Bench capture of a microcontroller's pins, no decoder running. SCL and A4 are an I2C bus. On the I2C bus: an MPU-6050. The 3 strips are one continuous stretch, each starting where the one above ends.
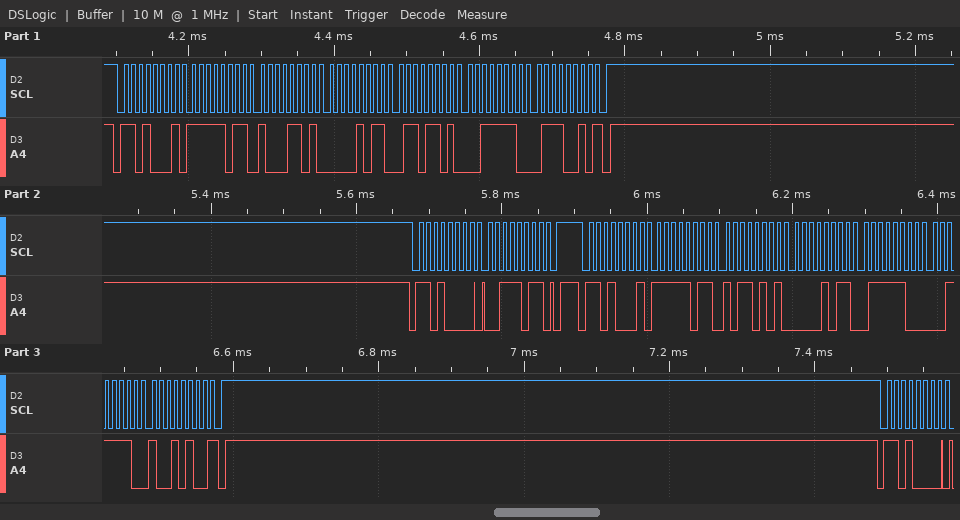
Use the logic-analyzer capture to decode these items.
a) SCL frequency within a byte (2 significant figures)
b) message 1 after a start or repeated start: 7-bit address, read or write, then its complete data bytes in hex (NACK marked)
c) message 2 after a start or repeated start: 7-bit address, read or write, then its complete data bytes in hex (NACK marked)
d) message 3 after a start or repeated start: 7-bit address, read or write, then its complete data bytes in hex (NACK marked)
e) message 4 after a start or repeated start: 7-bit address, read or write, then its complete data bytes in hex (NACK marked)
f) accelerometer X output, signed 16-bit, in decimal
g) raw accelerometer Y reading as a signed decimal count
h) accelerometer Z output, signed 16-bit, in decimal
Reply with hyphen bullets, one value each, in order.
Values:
- 100 kHz
- 0x68 read: FB 8D 0B 6D 3E 72 NACK
- 0x68 write: 3B
- 0x68 read: FB B5 0B 7C 3E 94 NACK
- 0x68 write
- -1099
- 2940
- 16020
